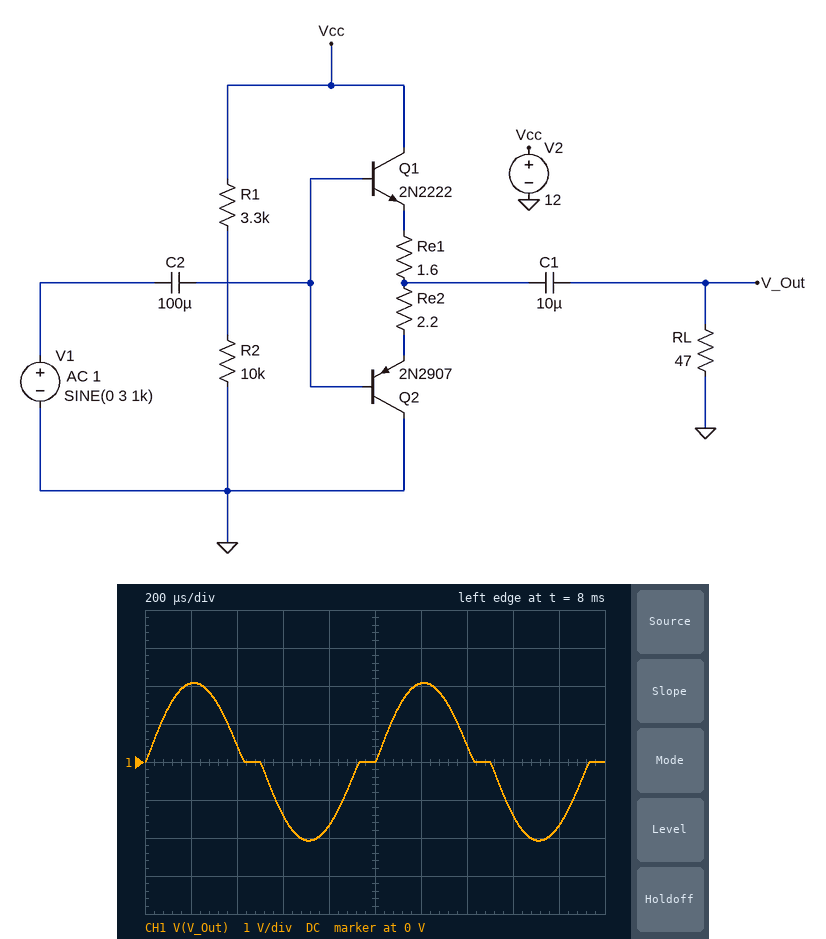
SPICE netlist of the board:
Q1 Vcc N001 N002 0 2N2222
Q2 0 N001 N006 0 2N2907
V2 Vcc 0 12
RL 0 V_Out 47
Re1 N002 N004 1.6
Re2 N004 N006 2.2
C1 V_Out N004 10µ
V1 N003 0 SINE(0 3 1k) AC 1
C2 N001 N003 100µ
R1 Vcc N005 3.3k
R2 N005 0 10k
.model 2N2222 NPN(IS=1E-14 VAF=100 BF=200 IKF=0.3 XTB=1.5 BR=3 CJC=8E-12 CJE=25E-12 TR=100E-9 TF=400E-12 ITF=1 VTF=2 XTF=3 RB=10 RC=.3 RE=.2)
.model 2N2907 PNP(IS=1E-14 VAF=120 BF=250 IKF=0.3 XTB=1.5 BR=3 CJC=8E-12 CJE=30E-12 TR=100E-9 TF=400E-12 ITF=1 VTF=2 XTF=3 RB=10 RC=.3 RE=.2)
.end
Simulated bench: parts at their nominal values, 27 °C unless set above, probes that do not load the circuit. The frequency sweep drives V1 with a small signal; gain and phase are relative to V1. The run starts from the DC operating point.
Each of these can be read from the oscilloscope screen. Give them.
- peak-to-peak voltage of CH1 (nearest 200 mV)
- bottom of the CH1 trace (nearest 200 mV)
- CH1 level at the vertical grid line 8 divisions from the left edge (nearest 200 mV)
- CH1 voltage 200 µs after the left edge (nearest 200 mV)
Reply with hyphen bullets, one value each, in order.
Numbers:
- 4.2 V
- -2.0 V
- -1.4 V
- 2.0 V
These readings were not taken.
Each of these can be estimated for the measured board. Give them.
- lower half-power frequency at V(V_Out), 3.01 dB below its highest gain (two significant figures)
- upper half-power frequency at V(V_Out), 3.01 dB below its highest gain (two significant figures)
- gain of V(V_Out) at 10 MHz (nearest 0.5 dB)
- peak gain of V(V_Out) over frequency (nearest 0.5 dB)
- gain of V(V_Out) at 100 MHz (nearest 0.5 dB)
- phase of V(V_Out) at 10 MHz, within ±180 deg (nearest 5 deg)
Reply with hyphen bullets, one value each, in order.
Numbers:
- 53 MHz
- 4.4 GHz
- -16.0 dB
- -1.0 dB
- -2.0 dB
- 80 deg
